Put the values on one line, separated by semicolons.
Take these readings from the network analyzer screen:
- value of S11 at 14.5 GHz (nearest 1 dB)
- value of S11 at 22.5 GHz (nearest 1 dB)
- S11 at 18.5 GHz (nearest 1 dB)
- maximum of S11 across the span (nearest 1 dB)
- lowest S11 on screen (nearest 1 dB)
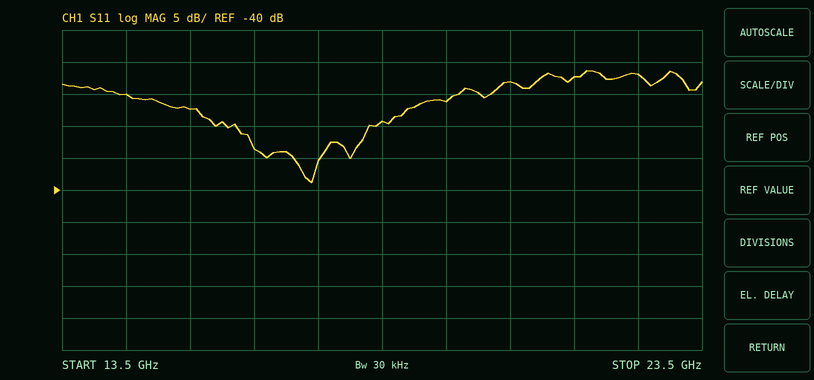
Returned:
-25 dB; -22 dB; -29 dB; -21 dB; -39 dB
